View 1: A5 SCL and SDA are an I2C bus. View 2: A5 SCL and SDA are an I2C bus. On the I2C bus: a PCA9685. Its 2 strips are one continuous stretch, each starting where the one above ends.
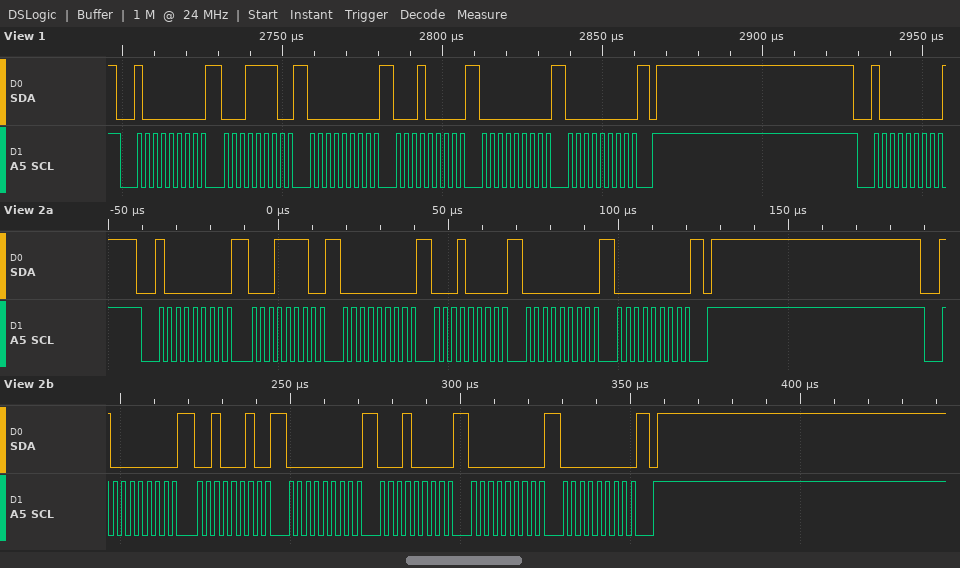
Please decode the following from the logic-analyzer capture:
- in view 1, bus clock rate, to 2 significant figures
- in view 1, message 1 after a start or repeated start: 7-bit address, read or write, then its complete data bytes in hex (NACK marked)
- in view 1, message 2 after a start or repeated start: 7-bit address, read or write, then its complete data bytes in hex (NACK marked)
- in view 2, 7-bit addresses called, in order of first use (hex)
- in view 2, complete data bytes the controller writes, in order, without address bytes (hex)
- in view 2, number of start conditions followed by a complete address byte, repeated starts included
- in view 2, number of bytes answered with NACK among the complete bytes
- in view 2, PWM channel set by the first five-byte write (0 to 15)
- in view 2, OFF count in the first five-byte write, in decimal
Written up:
400 kHz
0x40 write: 1E 00 10 00 00
0x40 write
0x40
1E 00 10 00 00 22 00 10 00 00
2
0
6
0
